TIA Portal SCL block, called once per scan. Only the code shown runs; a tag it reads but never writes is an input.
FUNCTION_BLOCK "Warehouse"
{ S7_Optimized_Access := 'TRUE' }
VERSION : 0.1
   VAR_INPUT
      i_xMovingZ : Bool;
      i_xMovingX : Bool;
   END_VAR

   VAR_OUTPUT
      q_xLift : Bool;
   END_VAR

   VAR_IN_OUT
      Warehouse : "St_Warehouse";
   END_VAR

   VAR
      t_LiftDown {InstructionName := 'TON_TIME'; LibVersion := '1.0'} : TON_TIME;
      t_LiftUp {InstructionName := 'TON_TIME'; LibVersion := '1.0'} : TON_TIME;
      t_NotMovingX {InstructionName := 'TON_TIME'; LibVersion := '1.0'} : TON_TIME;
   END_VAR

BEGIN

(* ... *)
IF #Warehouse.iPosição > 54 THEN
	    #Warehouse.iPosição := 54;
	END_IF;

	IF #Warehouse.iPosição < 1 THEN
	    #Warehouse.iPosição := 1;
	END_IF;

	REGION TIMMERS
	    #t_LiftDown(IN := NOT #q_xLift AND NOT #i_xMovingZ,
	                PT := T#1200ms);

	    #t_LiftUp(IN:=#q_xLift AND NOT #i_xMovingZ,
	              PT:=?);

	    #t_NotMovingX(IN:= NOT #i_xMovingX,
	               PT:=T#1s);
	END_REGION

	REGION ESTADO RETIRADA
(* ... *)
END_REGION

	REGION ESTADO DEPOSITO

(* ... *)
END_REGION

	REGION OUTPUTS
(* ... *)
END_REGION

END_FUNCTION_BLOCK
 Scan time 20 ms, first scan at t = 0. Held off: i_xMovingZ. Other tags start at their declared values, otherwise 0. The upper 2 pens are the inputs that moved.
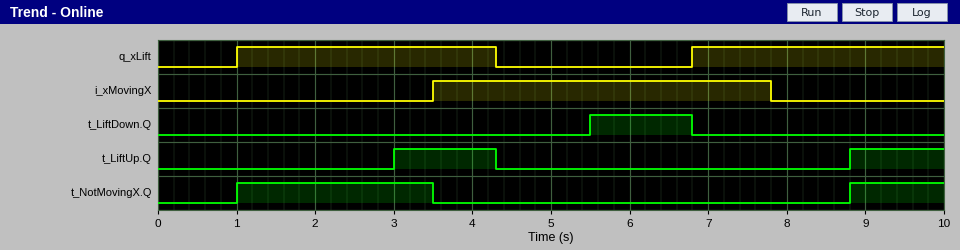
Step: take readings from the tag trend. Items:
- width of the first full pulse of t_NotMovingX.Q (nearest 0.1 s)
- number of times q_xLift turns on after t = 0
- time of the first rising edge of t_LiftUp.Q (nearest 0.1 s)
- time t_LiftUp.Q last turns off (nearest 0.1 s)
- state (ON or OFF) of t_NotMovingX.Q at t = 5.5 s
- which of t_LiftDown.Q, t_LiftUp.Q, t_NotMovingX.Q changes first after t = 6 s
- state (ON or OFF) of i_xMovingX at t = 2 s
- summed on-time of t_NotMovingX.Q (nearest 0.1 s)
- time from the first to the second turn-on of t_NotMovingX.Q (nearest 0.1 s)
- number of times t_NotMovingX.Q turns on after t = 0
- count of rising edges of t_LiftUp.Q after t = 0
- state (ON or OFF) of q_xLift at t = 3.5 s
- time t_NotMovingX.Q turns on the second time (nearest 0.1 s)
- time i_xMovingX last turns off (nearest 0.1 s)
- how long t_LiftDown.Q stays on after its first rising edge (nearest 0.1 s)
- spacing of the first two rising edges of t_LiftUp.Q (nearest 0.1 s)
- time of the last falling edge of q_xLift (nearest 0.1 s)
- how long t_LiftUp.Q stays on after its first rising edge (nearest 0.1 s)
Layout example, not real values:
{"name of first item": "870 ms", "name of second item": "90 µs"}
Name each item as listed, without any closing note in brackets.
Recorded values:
{"width of the first full pulse of t_NotMovingX.Q": "2.5 s", "number of times q_xLift turns on after t = 0": "2", "time of the first rising edge of t_LiftUp.Q": "3.0 s", "time t_LiftUp.Q last turns off": "4.3 s", "state (ON or OFF) of t_NotMovingX.Q at t = 5.5 s": "OFF", "which of t_LiftDown.Q, t_LiftUp.Q, t_NotMovingX.Q changes first after t = 6 s": "t_LiftDown.Q", "state (ON or OFF) of i_xMovingX at t = 2 s": "OFF", "summed on-time of t_NotMovingX.Q": "3.7 s", "time from the first to the second turn-on of t_NotMovingX.Q": "7.8 s", "number of times t_NotMovingX.Q turns on after t = 0": "2", "count of rising edges of t_LiftUp.Q after t = 0": "2", "state (ON or OFF) of q_xLift at t = 3.5 s": "ON", "time t_NotMovingX.Q turns on the second time": "8.8 s", "time i_xMovingX last turns off": "7.8 s", "how long t_LiftDown.Q stays on after its first rising edge": "1.3 s", "spacing of the first two rising edges of t_LiftUp.Q": "5.8 s", "time of the last falling edge of q_xLift": "4.3 s", "how long t_LiftUp.Q stays on after its first rising edge": "1.3 s"}
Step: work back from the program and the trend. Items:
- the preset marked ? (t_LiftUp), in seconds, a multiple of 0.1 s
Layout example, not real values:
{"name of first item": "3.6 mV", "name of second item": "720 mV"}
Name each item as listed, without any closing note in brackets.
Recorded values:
{"the preset marked ? (t_LiftUp), in seconds, a multiple of 0.1 s": "2.0 s"}
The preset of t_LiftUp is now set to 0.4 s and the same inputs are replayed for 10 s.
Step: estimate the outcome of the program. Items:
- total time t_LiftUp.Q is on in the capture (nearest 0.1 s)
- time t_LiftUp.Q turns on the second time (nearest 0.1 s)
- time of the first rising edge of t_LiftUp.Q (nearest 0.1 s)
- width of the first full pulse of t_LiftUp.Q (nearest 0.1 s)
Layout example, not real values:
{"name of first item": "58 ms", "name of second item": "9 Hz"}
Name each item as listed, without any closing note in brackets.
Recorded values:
{"total time t_LiftUp.Q is on in the capture": "5.7 s", "time t_LiftUp.Q turns on the second time": "7.2 s", "time of the first rising edge of t_LiftUp.Q": "1.4 s", "width of the first full pulse of t_LiftUp.Q": "2.9 s"}
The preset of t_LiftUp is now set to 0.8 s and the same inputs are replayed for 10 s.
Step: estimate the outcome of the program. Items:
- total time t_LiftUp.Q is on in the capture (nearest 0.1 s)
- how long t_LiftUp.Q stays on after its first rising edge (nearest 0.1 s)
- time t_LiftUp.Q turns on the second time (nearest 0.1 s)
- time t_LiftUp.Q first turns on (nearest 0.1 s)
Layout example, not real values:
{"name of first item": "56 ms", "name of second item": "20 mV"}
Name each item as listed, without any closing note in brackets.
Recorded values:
{"total time t_LiftUp.Q is on in the capture": "4.9 s", "how long t_LiftUp.Q stays on after its first rising edge": "2.5 s", "time t_LiftUp.Q turns on the second time": "7.6 s", "time t_LiftUp.Q first turns on": "1.8 s"}
